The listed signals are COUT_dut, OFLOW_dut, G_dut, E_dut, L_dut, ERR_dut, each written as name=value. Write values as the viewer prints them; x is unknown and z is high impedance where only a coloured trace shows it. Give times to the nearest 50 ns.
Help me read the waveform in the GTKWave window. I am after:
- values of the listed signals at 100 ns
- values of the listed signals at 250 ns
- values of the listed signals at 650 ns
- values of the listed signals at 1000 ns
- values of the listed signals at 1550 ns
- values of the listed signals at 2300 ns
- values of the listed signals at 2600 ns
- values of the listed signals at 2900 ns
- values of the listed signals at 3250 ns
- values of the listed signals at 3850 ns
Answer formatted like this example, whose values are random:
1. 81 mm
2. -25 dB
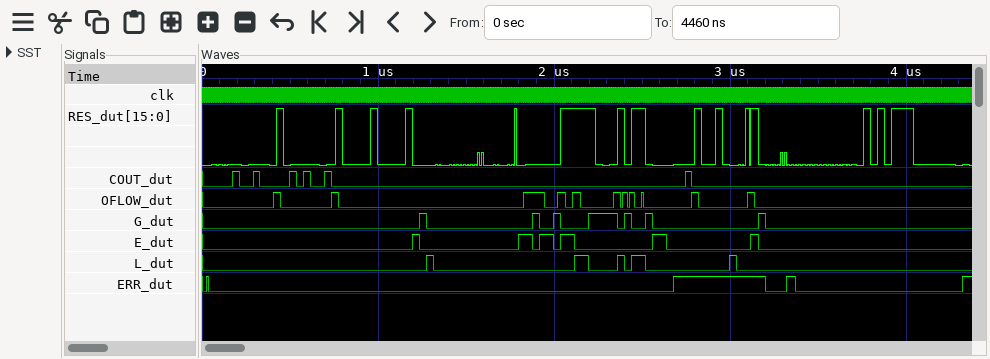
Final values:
1. COUT_dut=0, OFLOW_dut=0, G_dut=0, E_dut=0, L_dut=0, ERR_dut=0
2. COUT_dut=0, OFLOW_dut=0, G_dut=0, E_dut=0, L_dut=0, ERR_dut=0
3. COUT_dut=0, OFLOW_dut=0, G_dut=0, E_dut=0, L_dut=0, ERR_dut=0
4. COUT_dut=0, OFLOW_dut=0, G_dut=0, E_dut=0, L_dut=0, ERR_dut=0
5. COUT_dut=0, OFLOW_dut=0, G_dut=0, E_dut=0, L_dut=0, ERR_dut=0
6. COUT_dut=0, OFLOW_dut=0, G_dut=1, E_dut=0, L_dut=0, ERR_dut=0
7. COUT_dut=0, OFLOW_dut=0, G_dut=0, E_dut=1, L_dut=0, ERR_dut=0
8. COUT_dut=0, OFLOW_dut=0, G_dut=0, E_dut=0, L_dut=0, ERR_dut=1
9. COUT_dut=0, OFLOW_dut=0, G_dut=0, E_dut=0, L_dut=0, ERR_dut=0
10. COUT_dut=0, OFLOW_dut=0, G_dut=0, E_dut=0, L_dut=0, ERR_dut=0
